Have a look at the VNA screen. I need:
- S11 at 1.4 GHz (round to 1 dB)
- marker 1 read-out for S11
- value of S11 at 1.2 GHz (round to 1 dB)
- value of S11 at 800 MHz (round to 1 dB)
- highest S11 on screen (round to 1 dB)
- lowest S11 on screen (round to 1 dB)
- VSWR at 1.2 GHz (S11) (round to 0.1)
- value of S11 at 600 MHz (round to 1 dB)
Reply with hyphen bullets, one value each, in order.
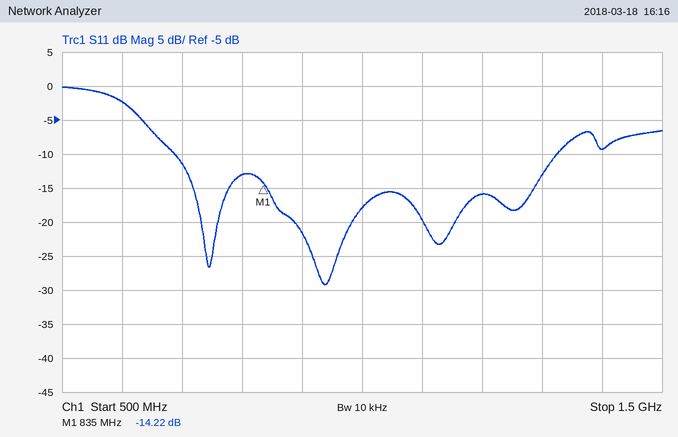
- -9 dB
- -14.22 dB
- -16 dB
- -13 dB
- 0 dB
- -29 dB
- 1.4
- -2 dB
